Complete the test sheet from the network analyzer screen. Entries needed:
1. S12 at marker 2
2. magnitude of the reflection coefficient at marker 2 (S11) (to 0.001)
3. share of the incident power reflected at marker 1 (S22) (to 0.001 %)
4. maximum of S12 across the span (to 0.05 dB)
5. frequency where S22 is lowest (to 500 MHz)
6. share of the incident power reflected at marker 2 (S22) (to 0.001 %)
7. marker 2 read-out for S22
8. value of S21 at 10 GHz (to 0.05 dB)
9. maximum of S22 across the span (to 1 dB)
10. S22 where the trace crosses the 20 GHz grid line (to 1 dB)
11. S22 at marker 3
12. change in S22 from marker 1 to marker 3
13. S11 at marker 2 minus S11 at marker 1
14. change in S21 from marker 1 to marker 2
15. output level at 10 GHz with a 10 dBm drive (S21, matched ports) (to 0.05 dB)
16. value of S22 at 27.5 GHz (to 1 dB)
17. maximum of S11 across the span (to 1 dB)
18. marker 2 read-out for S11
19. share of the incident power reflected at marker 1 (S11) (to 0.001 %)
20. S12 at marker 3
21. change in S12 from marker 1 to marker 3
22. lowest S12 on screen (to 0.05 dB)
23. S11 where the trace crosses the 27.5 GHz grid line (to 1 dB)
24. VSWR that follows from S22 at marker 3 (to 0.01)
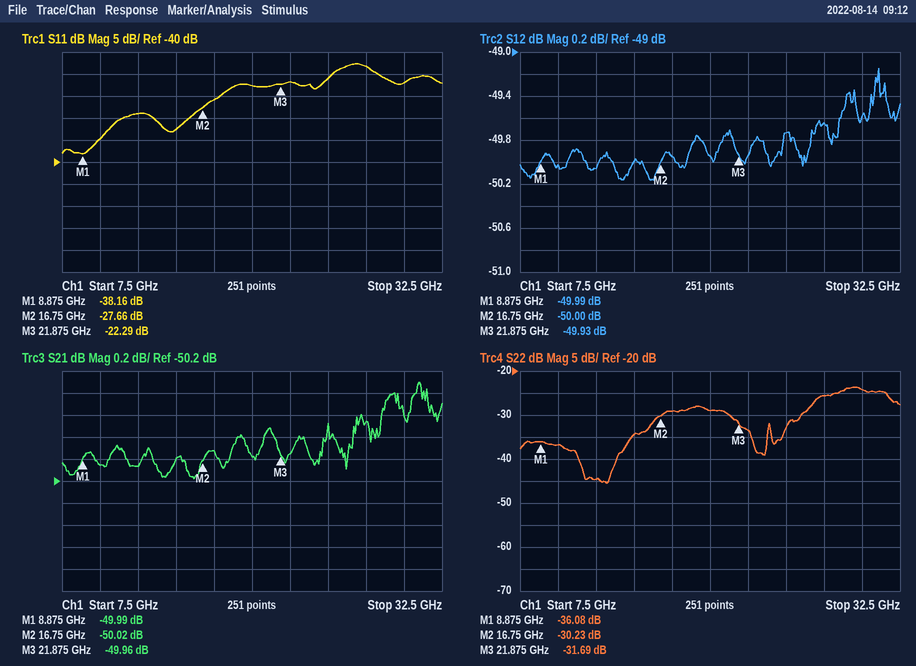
-50.00 dB
0.041
0.025 %
-49.15 dB
13.0 GHz
0.095 %
-30.23 dB
-50.05 dB
-24 dB
-29 dB
-31.69 dB
4.39 dB
10.50 dB
-0.03 dB
-40.05 dBm
-26 dB
-18 dB
-27.66 dB
0.015 %
-49.93 dB
0.06 dB
-50.15 dB
-18 dB
1.05
